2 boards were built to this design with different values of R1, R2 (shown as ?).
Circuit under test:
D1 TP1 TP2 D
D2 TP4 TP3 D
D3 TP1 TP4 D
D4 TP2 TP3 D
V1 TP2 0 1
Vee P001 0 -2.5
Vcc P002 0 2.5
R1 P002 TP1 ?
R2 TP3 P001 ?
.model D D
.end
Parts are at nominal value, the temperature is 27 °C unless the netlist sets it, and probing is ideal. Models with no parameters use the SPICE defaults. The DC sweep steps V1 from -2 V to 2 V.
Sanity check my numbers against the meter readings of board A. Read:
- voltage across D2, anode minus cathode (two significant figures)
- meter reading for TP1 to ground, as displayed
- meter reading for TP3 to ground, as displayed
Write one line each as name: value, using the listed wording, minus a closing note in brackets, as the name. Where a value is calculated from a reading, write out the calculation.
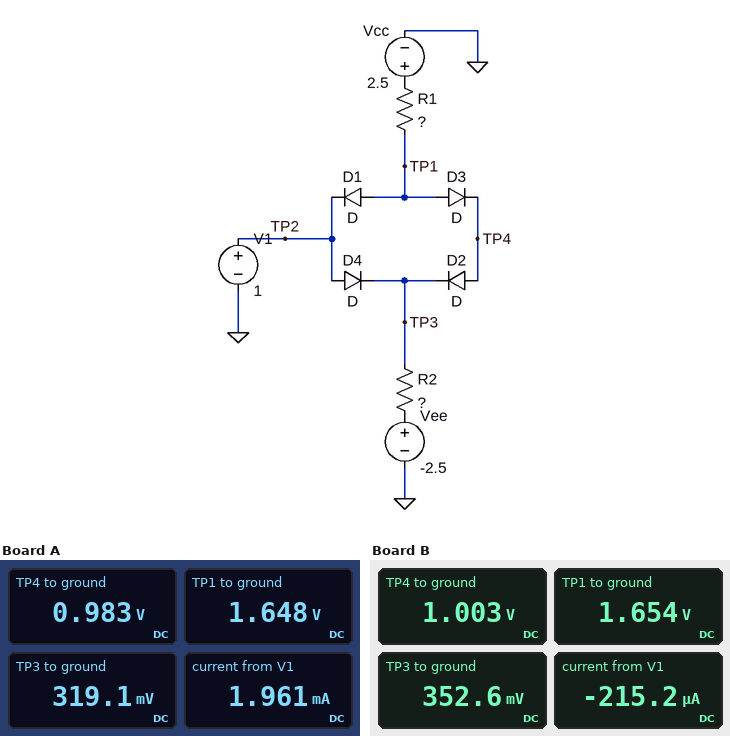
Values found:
voltage across D2, anode minus cathode: 983 mV - 319.1 mV = 660 mV
meter reading for TP1 to ground, as displayed: 1.648 V
meter reading for TP3 to ground, as displayed: 319.1 mV
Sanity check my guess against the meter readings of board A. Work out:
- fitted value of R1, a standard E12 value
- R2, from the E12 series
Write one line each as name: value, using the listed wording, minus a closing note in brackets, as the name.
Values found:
fitted value of R1, a standard E12 value: 390 Ω
R2, from the E12 series: 680 Ω
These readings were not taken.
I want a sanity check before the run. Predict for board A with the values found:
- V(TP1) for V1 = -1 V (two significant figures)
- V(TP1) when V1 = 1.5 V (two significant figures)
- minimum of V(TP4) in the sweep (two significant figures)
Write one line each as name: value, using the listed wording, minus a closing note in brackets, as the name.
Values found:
V(TP1) for V1 = -1 V: -300 mV
V(TP1) when V1 = 1.5 V: 2.1 V
minimum of V(TP4) in the sweep: -1.9 V
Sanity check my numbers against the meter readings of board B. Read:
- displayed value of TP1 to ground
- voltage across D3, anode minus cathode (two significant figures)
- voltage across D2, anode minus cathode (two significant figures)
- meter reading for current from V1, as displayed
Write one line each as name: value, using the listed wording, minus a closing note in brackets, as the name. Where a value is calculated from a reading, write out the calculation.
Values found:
displayed value of TP1 to ground: 1.654 V
voltage across D3, anode minus cathode: 1.654 V - 1.003 V = 650 mV
voltage across D2, anode minus cathode: 1.003 V - 352.6 mV = 650 mV
meter reading for current from V1, as displayed: -215.2 µA
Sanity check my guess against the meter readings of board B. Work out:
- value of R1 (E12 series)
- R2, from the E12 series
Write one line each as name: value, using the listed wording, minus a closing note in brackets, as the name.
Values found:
value of R1: 470 Ω
R2, from the E12 series: 1.8 kΩ
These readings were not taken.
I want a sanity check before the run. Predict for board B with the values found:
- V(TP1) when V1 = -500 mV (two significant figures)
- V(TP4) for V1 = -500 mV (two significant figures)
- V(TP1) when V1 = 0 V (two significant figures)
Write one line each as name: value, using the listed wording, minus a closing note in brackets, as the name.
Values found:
V(TP1) when V1 = -500 mV: 190 mV
V(TP4) for V1 = -500 mV: -450 mV
V(TP1) when V1 = 0 V: 680 mV
